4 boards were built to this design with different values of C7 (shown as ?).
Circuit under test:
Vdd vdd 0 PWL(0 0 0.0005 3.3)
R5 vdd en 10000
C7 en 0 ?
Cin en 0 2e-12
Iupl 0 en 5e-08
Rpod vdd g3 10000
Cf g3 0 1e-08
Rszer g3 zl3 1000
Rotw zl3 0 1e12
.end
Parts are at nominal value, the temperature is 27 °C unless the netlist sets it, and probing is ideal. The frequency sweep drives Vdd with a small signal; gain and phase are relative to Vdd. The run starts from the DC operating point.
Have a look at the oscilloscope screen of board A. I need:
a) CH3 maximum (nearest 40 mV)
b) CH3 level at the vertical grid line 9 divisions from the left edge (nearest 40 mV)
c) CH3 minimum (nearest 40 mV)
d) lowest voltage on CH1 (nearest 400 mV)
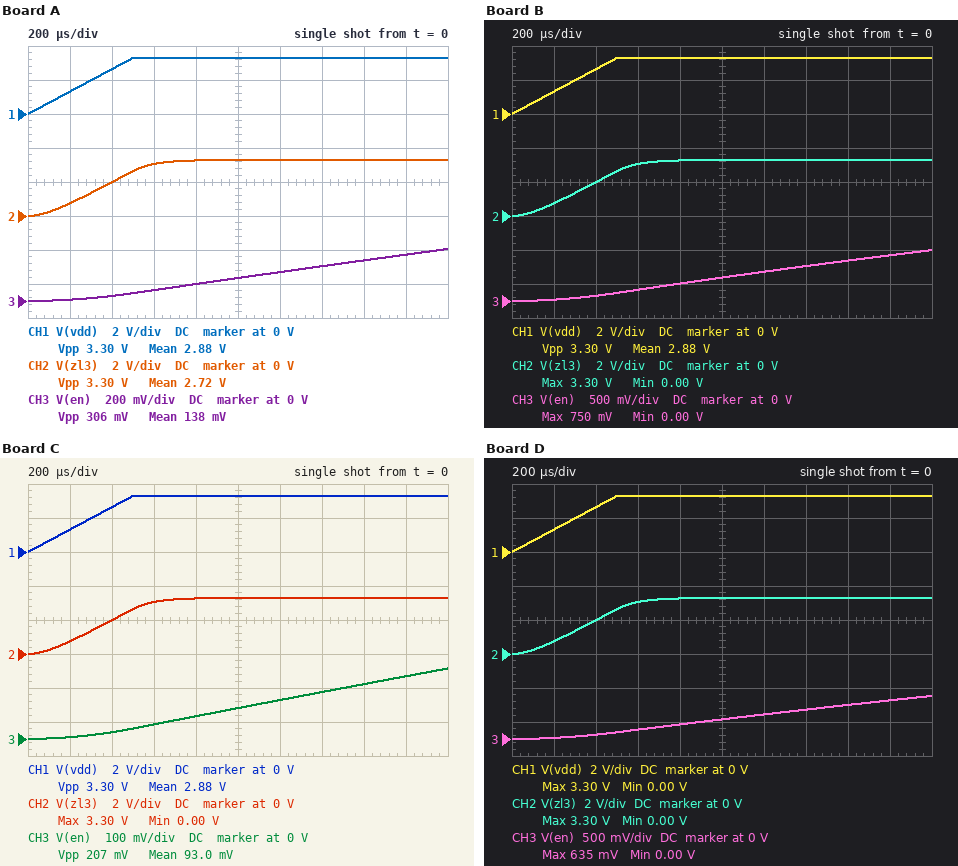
320 mV
280 mV
0 V
0 V
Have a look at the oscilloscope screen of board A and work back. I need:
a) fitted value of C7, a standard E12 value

1.8 µF
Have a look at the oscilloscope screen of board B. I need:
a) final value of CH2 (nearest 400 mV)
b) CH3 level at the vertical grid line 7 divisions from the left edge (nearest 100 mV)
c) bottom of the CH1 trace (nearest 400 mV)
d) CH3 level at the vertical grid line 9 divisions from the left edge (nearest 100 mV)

3.2 V
500 mV
0 V
700 mV
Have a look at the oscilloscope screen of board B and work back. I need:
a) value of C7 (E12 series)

680 nF
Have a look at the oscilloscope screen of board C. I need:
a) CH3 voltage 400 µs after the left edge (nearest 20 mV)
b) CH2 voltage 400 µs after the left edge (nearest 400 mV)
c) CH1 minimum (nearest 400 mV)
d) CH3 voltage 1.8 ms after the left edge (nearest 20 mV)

20 mV
2.0 V
0 V
180 mV
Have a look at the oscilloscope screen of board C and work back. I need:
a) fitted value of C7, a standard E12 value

2.7 µF
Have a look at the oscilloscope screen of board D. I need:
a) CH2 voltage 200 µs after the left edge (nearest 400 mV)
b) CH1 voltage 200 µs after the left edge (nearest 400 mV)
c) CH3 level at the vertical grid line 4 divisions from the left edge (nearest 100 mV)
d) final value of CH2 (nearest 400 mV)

800 mV
1.2 V
200 mV
3.2 V
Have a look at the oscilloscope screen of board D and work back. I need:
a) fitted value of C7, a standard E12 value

820 nF
